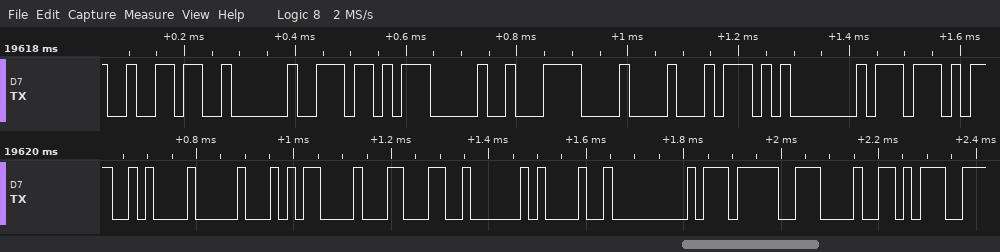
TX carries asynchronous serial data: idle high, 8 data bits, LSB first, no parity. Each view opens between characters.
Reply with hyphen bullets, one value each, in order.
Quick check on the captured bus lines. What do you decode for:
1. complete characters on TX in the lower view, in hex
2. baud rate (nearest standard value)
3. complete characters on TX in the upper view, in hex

- 0A, 10, 0D, 8C, 02, 21, 00, F7, 0E, D6
- 57600 baud
- B2, 02, 6E, 07, E2, 08, 74, 01, 77
